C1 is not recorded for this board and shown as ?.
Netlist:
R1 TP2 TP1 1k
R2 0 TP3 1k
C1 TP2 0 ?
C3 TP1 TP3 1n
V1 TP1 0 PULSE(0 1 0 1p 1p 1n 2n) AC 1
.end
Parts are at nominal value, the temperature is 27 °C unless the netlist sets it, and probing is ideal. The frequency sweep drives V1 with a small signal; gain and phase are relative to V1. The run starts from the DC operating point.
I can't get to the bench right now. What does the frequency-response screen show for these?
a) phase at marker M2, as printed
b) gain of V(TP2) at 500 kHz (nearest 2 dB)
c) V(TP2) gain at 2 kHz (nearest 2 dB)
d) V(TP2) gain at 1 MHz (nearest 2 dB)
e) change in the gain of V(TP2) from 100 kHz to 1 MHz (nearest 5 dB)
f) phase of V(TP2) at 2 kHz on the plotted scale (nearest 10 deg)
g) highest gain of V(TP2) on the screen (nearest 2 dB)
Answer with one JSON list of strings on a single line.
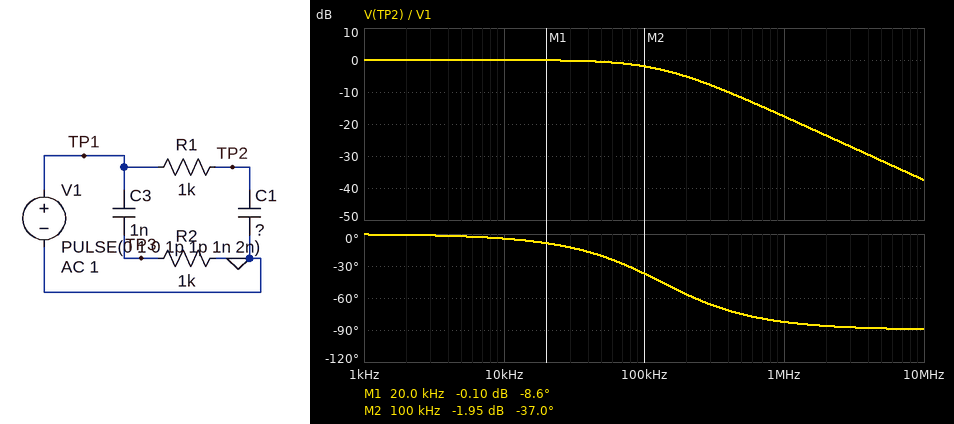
["-37.0 deg", "-12 dB", "0 dB", "-18 dB", "-15 dB", "0 deg", "0 dB"]
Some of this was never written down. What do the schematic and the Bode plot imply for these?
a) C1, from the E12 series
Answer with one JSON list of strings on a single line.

["1.2 nF"]
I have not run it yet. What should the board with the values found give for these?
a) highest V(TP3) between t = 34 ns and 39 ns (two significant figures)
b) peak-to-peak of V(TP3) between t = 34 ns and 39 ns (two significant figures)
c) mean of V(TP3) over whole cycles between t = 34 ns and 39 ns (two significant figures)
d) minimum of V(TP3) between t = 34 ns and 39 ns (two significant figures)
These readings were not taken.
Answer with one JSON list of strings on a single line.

["980 mV", "1.0 V", "480 mV", "-19 mV"]
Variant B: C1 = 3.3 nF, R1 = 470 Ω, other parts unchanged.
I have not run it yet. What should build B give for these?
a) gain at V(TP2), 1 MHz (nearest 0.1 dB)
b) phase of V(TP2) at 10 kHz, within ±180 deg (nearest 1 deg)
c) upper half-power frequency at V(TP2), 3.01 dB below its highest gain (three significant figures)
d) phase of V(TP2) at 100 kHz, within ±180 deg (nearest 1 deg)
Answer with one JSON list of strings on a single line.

["-19.8 dB", "-6 deg", "103 kHz", "-44 deg"]
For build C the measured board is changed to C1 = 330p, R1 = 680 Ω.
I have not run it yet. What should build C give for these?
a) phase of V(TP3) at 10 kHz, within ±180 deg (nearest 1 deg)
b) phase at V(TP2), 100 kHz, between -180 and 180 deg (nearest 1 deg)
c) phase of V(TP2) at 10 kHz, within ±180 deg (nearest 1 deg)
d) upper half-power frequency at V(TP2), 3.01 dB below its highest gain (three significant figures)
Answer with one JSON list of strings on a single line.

["86 deg", "-8 deg", "-1 deg", "709 kHz"]
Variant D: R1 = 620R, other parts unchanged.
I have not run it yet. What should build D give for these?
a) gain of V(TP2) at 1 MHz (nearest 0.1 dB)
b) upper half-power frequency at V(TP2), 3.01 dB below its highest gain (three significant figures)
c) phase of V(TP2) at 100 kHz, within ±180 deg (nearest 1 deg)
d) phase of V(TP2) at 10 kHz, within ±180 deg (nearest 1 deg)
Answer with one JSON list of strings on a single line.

["-13.6 dB", "214 kHz", "-25 deg", "-3 deg"]
